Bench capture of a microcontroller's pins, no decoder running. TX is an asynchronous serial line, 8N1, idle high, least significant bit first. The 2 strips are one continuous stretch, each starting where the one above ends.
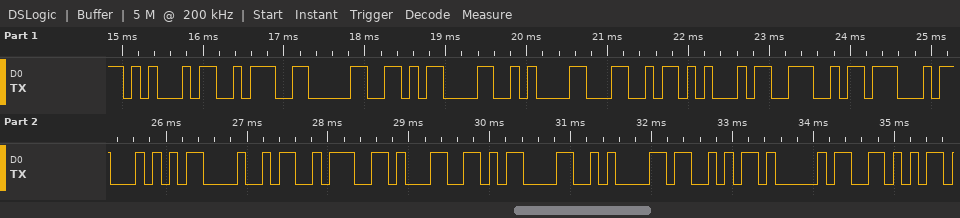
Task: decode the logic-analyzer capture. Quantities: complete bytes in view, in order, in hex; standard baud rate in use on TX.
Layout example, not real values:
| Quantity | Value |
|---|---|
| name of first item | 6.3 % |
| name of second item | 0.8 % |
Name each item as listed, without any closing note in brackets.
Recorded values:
| Quantity | Value |
|---|---|
| complete bytes in view, in order, in hex | 0x45 0x3A 0x30 0x0D 0x0A 0x4C 0x45 0x4E 0x47 0x54 0x48 0x3A 0x31 0x0D 0x0A 0x53 0x41 0x56 |
| standard baud rate in use on TX | 9600 baud |
